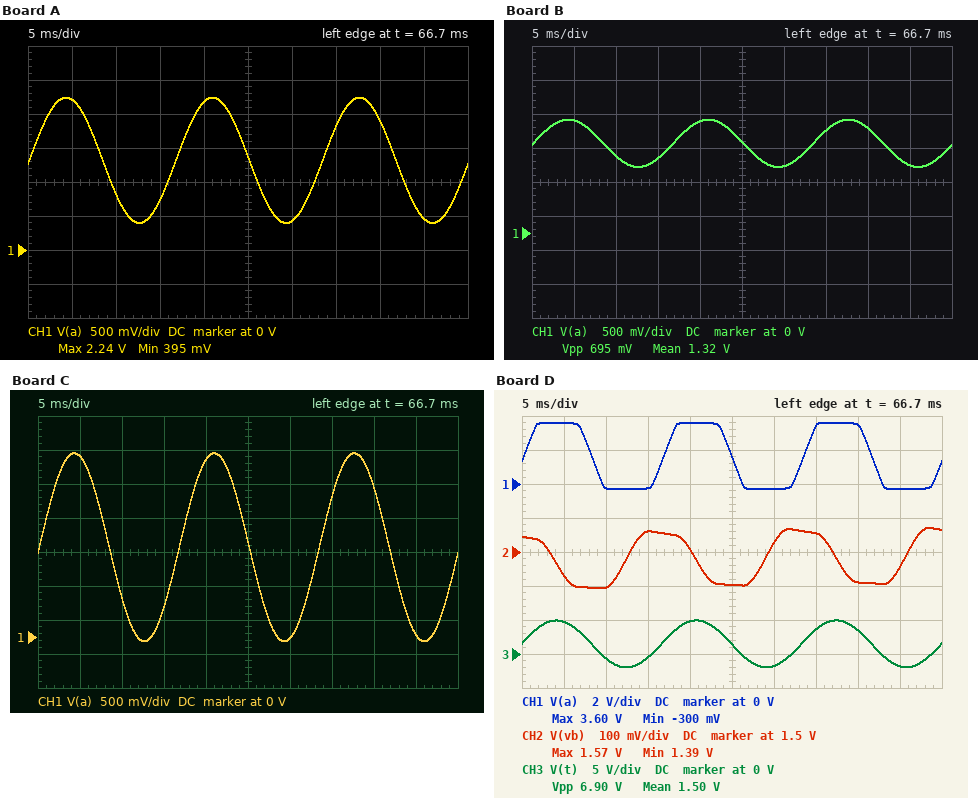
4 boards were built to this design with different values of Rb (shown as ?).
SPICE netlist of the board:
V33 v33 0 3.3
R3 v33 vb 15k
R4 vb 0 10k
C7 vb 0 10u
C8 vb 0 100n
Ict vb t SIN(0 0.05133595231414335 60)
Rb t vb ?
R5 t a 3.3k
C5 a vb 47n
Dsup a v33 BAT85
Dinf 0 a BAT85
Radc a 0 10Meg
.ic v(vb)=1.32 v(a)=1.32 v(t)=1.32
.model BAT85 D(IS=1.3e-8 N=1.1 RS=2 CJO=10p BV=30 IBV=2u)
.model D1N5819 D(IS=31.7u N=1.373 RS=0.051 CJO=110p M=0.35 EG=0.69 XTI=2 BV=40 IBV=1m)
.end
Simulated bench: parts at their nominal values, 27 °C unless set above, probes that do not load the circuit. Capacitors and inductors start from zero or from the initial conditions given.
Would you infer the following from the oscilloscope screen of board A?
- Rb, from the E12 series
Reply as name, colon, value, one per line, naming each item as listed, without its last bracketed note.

Rb, from the E12 series: 18 Ω
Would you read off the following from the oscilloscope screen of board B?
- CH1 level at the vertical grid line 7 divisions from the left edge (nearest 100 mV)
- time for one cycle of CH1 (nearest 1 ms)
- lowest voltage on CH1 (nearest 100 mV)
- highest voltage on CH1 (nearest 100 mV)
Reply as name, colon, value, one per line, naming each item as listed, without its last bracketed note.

CH1 level at the vertical grid line 7 divisions from the left edge: 1.5 V
time for one cycle of CH1: 17 ms
lowest voltage on CH1: 1.0 V
highest voltage on CH1: 1.7 V
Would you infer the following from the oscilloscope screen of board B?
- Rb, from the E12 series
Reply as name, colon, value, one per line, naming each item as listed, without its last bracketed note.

Rb, from the E12 series: 6.8 Ω
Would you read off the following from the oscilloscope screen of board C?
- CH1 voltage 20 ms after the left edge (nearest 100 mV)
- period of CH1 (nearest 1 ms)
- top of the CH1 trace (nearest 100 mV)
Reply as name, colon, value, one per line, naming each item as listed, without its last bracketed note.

CH1 voltage 20 ms after the left edge: 2.6 V
period of CH1: 17 ms
top of the CH1 trace: 2.7 V
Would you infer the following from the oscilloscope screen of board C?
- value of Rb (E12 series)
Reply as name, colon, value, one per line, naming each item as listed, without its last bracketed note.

value of Rb: 27 Ω
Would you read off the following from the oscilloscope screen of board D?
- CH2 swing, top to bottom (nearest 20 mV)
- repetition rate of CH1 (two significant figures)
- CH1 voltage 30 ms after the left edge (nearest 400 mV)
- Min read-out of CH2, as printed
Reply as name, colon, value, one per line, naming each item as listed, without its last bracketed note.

CH2 swing, top to bottom: 180 mV
repetition rate of CH1: 60 Hz
CH1 voltage 30 ms after the left edge: -400 mV
Min read-out of CH2, as printed: 1.39 V
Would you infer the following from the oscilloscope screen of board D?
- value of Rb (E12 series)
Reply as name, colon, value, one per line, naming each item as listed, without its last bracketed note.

value of Rb: 68 Ω
